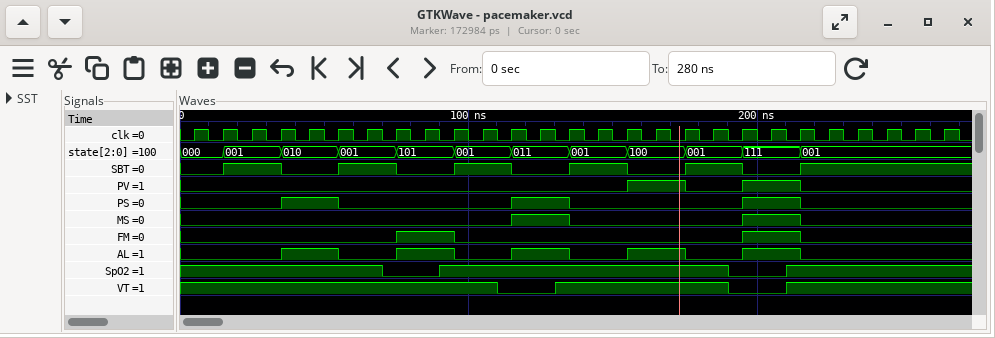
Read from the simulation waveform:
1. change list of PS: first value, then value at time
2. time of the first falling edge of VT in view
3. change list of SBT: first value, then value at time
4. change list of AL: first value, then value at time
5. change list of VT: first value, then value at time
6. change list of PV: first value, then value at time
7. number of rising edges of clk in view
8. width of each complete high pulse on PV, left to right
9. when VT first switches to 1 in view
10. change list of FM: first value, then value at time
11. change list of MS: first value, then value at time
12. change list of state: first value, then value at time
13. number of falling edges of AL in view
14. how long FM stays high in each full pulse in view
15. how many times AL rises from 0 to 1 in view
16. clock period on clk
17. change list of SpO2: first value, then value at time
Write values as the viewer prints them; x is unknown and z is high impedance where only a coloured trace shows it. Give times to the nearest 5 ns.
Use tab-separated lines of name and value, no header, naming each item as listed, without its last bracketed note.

change list of PS: first value, then value at time	0, 1 at 35 ns, 0 at 55 ns, 1 at 115 ns, 0 at 135 ns, 1 at 195 ns, 0 at 215 ns
time of the first falling edge of VT in view	110 ns
change list of SBT: first value, then value at time	0, 1 at 15 ns, 0 at 35 ns, 1 at 55 ns, 0 at 75 ns, 1 at 95 ns, 0 at 115 ns, 1 at 135 ns, 0 at 155 ns, 1 at 175 ns, 0 at 195 ns, 1 at 215 ns
change list of AL: first value, then value at time	0, 1 at 35 ns, 0 at 55 ns, 1 at 75 ns, 0 at 95 ns, 1 at 115 ns, 0 at 135 ns, 1 at 155 ns, 0 at 175 ns, 1 at 195 ns, 0 at 215 ns
change list of VT: first value, then value at time	1, 0 at 110 ns, 1 at 130 ns, 0 at 190 ns, 1 at 210 ns
change list of PV: first value, then value at time	0, 1 at 155 ns, 0 at 175 ns, 1 at 195 ns, 0 at 215 ns
number of rising edges of clk in view	27
width of each complete high pulse on PV, left to right	20 ns, 20 ns
when VT first switches to 1 in view	130 ns
change list of FM: first value, then value at time	0, 1 at 75 ns, 0 at 95 ns, 1 at 195 ns, 0 at 215 ns
change list of MS: first value, then value at time	0, 1 at 115 ns, 0 at 135 ns, 1 at 195 ns, 0 at 215 ns
change list of state: first value, then value at time	000, 001 at 15 ns, 010 at 35 ns, 001 at 55 ns, 101 at 75 ns, 001 at 95 ns, 011 at 115 ns, 001 at 135 ns, 100 at 155 ns, 001 at 175 ns, 111 at 195 ns, 001 at 215 ns
number of falling edges of AL in view	5
how long FM stays high in each full pulse in view	20 ns, 20 ns
how many times AL rises from 0 to 1 in view	5
clock period on clk	10 ns
change list of SpO2: first value, then value at time	1, 0 at 70 ns, 1 at 90 ns, 0 at 190 ns, 1 at 210 ns
